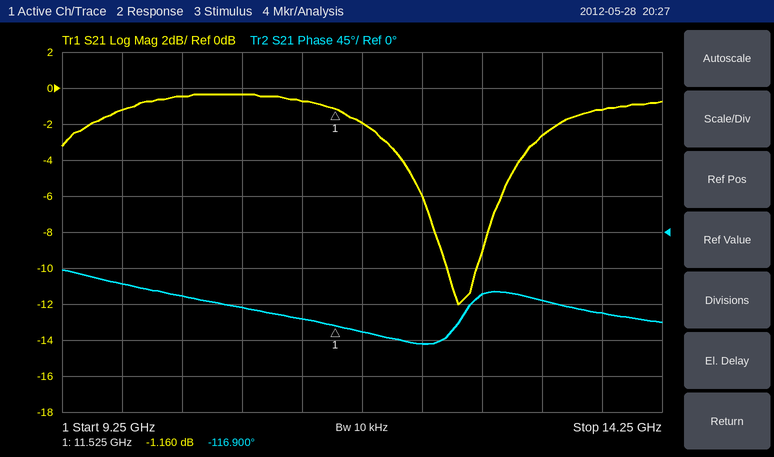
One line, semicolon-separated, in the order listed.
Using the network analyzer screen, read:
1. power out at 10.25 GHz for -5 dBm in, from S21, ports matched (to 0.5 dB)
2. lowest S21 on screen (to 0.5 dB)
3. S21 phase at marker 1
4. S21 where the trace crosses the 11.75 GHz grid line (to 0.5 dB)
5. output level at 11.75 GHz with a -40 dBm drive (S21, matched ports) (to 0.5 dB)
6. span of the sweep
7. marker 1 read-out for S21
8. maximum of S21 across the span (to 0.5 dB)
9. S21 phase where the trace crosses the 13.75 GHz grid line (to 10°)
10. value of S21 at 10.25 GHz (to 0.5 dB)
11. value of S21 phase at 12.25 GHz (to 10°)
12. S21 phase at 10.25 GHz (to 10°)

-5.5 dBm; -12.0 dB; -116.900°; -2.0 dB; -42.0 dBm; 5 GHz; -1.160 dB; -0.5 dB; -100°; -0.5 dB; -140°; -80°
